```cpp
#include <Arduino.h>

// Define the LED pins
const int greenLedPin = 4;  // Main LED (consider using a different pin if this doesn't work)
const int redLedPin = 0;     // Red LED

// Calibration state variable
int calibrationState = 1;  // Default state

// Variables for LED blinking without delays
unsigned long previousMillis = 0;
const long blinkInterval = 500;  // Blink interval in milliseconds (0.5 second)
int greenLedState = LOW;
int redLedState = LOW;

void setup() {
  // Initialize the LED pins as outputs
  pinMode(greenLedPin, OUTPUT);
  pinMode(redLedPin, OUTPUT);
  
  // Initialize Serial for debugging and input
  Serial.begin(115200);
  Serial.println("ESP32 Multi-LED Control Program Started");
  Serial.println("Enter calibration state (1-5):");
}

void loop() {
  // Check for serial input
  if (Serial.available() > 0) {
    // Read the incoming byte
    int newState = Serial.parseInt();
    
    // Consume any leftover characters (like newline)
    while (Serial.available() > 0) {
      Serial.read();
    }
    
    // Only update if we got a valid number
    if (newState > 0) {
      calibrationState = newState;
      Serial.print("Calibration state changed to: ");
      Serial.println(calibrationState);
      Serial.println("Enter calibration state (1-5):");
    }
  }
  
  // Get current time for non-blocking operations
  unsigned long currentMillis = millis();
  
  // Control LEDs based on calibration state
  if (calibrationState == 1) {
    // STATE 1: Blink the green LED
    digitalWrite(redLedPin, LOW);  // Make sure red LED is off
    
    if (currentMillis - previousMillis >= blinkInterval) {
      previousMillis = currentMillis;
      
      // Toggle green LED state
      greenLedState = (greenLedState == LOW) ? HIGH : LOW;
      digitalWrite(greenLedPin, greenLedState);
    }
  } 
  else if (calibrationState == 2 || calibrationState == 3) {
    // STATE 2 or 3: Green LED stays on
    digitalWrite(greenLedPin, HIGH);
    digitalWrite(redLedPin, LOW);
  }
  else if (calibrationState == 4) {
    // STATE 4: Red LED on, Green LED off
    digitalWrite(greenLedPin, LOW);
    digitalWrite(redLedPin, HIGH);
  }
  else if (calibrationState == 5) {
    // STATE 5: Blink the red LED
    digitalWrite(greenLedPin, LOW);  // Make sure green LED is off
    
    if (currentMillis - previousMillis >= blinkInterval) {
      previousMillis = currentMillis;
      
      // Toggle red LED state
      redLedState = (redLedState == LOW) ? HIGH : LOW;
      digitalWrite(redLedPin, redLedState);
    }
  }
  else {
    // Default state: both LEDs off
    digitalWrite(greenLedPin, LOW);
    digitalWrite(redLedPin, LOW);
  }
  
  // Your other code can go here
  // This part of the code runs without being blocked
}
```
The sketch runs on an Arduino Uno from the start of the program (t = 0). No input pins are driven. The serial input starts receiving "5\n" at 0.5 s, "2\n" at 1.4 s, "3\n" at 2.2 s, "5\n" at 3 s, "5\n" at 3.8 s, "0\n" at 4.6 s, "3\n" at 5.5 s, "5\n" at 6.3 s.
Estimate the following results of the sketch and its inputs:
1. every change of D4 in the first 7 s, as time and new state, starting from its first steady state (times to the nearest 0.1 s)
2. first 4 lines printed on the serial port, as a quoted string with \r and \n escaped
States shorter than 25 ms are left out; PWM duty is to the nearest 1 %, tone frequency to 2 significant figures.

0 s low; 1.4 s high; 3 s low; 5.5 s high; 6.3 s low
"ESP32 Multi-LED Control Program Started\r\nEnter calibration state (1-5):\r\nCalibration state changed to: 5\r\nEnter calibration state (1-5):\r\n"
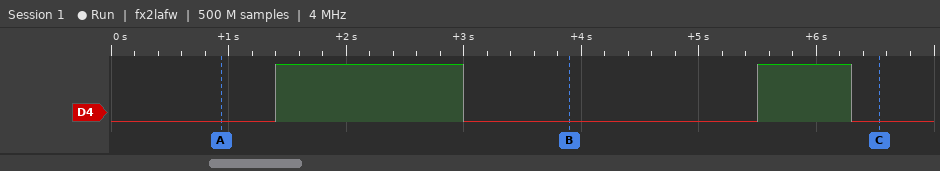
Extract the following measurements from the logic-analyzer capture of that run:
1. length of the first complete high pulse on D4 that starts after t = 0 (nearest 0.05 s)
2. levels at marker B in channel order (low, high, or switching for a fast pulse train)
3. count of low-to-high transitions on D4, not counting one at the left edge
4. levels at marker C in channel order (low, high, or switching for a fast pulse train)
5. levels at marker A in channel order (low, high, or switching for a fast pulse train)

1.60 s
D4 low
2
D4 low
D4 low
